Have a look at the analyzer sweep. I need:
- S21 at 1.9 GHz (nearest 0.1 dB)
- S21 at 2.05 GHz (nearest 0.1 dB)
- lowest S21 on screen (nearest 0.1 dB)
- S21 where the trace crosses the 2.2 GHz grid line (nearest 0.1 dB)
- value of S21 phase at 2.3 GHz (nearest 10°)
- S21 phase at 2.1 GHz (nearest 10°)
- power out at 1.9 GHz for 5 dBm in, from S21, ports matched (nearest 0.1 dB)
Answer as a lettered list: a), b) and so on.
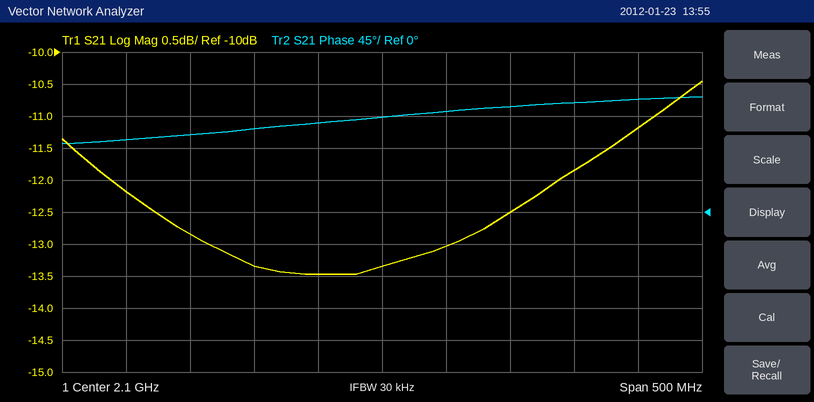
a) -12.2 dB
b) -13.5 dB
c) -13.5 dB
d) -12.5 dB
e) 160°
f) 130°
g) -7.2 dBm
